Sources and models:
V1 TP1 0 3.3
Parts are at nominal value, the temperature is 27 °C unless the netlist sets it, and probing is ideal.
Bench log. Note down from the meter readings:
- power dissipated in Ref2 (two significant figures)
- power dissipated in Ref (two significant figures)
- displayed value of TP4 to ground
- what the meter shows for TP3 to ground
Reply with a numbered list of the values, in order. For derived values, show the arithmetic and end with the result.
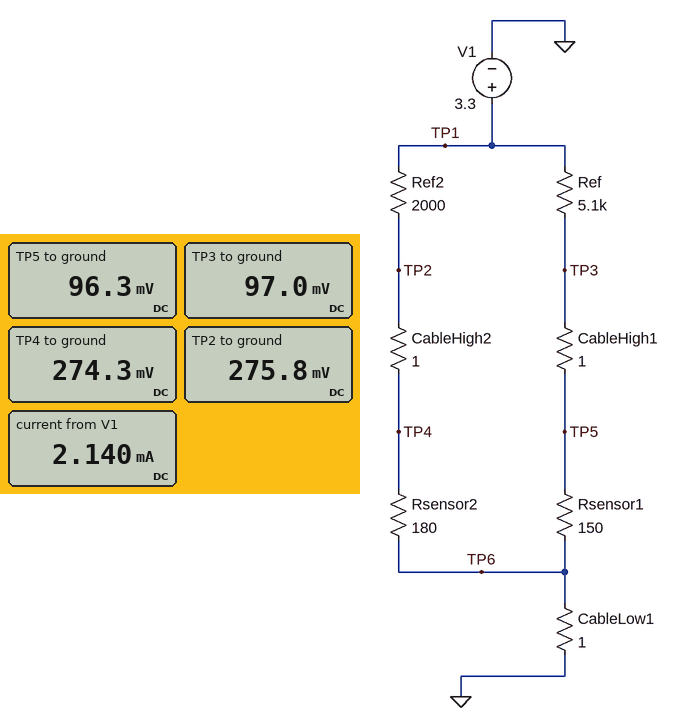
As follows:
1. (3.3 V - 275.8 mV)^2 / 2 kΩ = 4.6 mW
2. (3.3 V - 97 mV)^2 / 5.1 kΩ = 2.0 mW
3. 274.3 mV
4. 97.0 mV
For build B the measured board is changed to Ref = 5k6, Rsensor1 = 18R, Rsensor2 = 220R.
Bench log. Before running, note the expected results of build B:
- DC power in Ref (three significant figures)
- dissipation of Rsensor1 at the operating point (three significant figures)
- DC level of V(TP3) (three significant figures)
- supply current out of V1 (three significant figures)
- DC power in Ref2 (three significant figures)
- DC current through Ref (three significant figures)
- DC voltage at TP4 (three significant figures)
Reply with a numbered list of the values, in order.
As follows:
1. 1.93 mW
2. 6.20 µW
3. 13.2 mV
4. 2.07 mA
5. 4.41 mW
6. 587 µA
7. 329 mV
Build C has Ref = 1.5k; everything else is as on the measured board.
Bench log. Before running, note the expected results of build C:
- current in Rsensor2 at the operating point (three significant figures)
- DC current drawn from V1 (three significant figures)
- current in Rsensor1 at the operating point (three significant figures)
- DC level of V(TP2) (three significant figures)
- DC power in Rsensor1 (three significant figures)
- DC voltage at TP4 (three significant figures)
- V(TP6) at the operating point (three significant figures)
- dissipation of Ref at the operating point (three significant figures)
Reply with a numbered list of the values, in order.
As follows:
1. 1.51 mA
2. 3.51 mA
3. 2.00 mA
4. 277 mV
5. 598 µW
6. 276 mV
7. 3.51 mV
8. 5.98 mW
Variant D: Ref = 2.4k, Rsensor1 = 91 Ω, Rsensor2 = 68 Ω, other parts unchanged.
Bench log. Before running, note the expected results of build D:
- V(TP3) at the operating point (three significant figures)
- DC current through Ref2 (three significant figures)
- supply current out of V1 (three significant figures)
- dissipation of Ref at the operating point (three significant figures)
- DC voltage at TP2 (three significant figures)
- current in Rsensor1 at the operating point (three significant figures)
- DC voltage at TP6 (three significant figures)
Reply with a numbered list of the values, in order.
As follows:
1. 125 mV
2. 1.59 mA
3. 2.92 mA
4. 4.20 mW
5. 113 mV
6. 1.32 mA
7. 2.92 mV
